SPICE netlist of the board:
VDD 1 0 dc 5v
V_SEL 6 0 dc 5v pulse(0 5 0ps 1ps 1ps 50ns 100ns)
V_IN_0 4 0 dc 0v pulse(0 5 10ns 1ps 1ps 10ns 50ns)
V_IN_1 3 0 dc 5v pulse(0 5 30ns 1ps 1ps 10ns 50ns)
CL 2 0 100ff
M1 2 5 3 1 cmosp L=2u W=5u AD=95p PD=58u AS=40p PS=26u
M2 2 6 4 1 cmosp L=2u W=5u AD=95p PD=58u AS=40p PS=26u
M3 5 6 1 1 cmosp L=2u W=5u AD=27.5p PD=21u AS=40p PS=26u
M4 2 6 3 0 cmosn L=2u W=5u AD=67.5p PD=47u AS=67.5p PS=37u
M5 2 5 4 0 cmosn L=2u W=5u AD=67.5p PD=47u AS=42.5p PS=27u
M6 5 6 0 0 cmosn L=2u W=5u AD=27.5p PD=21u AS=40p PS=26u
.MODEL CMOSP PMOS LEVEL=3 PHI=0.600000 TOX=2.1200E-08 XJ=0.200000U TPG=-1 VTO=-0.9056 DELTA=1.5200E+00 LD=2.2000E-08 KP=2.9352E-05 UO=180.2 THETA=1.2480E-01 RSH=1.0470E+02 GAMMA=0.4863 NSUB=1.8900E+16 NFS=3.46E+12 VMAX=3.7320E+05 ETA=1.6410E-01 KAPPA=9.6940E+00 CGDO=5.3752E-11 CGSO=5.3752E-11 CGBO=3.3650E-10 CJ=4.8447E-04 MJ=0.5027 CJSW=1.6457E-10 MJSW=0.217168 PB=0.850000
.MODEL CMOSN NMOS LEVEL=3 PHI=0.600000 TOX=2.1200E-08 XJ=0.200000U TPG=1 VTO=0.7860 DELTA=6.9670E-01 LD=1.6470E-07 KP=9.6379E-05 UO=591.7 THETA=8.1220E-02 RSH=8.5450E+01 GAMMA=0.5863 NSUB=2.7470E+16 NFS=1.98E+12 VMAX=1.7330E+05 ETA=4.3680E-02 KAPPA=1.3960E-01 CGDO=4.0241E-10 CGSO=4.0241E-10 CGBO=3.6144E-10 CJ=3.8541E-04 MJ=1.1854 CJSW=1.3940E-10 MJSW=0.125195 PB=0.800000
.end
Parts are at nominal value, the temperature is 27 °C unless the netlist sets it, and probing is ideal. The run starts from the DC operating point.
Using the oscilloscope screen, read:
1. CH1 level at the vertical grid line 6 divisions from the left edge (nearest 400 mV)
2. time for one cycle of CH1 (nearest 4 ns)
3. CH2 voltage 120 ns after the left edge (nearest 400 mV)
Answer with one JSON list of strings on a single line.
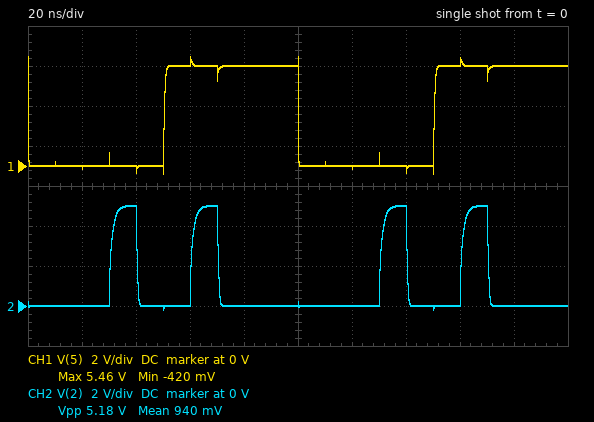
["0 V", "100 ns", "0 V"]
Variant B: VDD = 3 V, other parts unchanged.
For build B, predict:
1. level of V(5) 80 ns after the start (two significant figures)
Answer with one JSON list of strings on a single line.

["3.0 V"]
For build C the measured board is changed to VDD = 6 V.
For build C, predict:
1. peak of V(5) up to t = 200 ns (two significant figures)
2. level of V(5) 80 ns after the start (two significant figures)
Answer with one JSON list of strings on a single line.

["6.5 V", "6.0 V"]
